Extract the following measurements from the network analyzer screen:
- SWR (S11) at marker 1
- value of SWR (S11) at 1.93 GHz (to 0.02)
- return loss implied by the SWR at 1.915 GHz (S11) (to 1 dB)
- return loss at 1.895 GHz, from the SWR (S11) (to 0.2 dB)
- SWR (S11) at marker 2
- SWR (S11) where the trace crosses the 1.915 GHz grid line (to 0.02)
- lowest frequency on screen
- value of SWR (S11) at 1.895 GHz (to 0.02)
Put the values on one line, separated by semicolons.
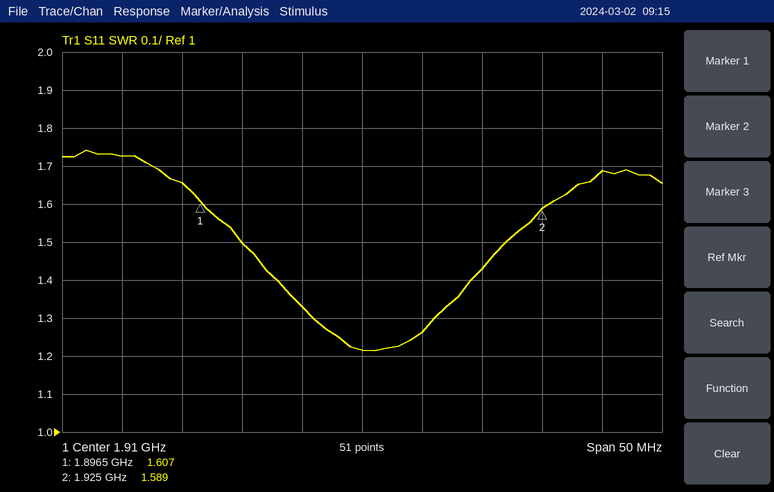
1.607; 1.68; 19 dB; 12.2 dB; 1.589; 1.26; 1.885 GHz; 1.66
